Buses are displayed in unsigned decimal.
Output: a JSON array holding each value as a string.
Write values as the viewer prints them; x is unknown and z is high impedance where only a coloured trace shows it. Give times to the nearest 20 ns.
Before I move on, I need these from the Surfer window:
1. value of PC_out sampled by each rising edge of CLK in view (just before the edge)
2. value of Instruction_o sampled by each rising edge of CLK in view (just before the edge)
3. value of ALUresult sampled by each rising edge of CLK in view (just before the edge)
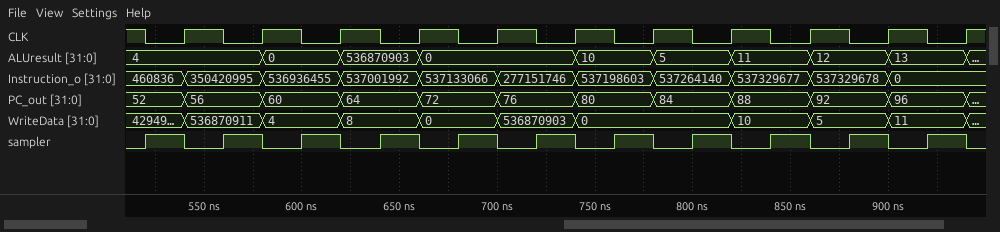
["52, 56, 60, 64, 72, 76, 80, 84, 88, 92, 96", "460836, 350420995, 536936455, 537001992, 537133066, 277151746, 537198603, 537264140, 537329677, 537329678, 0", "4, 4, 0, 536870903, 0, 0, 10, 5, 11, 12, 13"]
